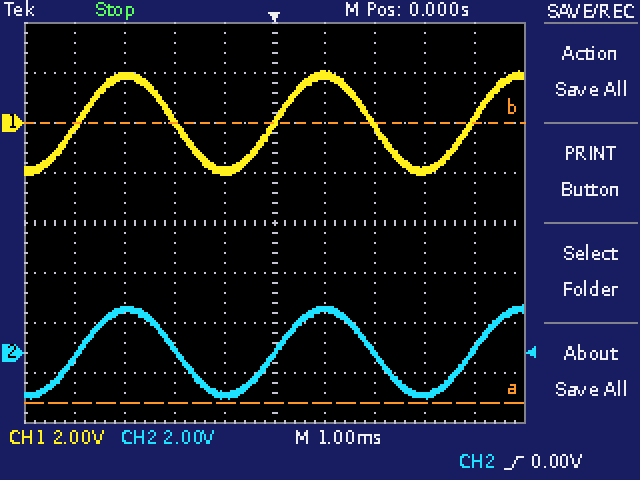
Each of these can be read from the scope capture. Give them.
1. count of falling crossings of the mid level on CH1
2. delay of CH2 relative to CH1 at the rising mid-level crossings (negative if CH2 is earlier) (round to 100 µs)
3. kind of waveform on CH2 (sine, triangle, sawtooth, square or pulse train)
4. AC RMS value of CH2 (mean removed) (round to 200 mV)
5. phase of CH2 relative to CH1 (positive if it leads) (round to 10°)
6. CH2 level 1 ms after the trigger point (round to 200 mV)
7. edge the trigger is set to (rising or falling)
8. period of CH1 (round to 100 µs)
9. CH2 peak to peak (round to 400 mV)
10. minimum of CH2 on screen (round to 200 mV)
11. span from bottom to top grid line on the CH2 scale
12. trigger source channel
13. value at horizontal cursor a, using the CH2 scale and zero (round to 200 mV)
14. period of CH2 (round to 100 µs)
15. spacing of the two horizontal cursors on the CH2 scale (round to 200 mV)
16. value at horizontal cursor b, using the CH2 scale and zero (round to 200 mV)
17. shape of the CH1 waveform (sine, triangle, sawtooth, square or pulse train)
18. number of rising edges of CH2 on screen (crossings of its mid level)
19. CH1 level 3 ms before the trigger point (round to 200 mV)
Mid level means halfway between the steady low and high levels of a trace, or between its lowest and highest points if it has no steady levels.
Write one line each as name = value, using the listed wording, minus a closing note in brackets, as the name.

count of falling crossings of the mid level on CH1 = 2
delay of CH2 relative to CH1 at the rising mid-level crossings (negative if CH2 is earlier) = 0.0 ms
kind of waveform on CH2 = sine
AC RMS value of CH2 (mean removed) = 1.2 V
phase of CH2 relative to CH1 (positive if it leads) = 0°
CH2 level 1 ms after the trigger point = 1.8 V
edge the trigger is set to = rising
period of CH1 = 3.9 ms
CH2 peak to peak = 3.6 V
minimum of CH2 on screen = -1.8 V
span from bottom to top grid line on the CH2 scale = 16 V
trigger source channel = CH2
value at horizontal cursor a, using the CH2 scale and zero = -2.0 V
period of CH2 = 3.9 ms
spacing of the two horizontal cursors on the CH2 scale = 11.2 V
value at horizontal cursor b, using the CH2 scale and zero = 9.2 V
shape of the CH1 waveform = sine
number of rising edges of CH2 on screen = 3
CH1 level 3 ms before the trigger point = 1.8 V
